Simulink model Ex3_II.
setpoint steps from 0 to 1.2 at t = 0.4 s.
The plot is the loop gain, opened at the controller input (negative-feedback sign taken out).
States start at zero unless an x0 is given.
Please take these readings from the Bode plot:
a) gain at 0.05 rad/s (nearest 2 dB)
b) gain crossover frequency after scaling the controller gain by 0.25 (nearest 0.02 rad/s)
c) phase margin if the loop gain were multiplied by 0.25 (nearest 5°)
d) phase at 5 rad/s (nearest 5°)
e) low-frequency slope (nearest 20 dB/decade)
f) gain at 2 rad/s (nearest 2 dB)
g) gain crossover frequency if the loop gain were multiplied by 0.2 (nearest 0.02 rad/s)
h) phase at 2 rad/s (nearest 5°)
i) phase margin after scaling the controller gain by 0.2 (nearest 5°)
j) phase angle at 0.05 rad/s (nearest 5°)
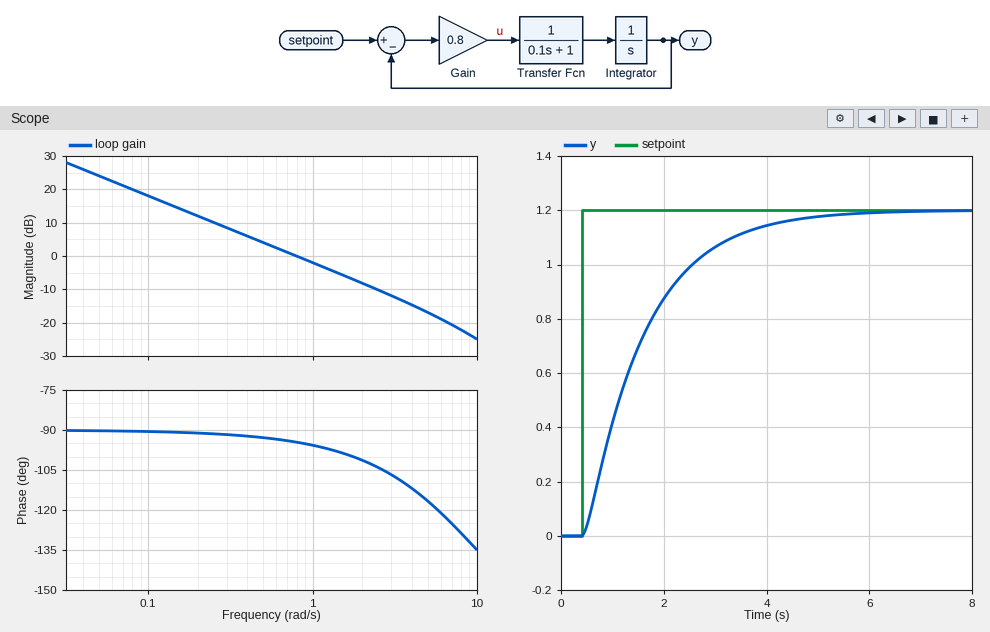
24 dB
0.20 rad/s
90°
-115°
-20 dB/decade
-8 dB
0.16 rad/s
-100°
90°
-90°
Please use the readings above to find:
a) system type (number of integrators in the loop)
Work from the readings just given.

1
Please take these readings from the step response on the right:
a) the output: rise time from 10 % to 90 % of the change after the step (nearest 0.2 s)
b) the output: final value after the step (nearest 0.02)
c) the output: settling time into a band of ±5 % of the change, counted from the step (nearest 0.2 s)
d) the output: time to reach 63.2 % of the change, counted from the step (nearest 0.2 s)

2.6 s
1.20
3.6 s
1.2 s
